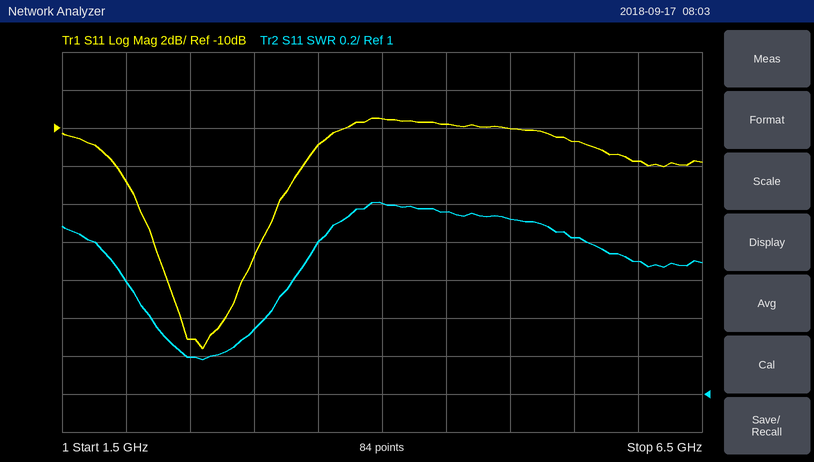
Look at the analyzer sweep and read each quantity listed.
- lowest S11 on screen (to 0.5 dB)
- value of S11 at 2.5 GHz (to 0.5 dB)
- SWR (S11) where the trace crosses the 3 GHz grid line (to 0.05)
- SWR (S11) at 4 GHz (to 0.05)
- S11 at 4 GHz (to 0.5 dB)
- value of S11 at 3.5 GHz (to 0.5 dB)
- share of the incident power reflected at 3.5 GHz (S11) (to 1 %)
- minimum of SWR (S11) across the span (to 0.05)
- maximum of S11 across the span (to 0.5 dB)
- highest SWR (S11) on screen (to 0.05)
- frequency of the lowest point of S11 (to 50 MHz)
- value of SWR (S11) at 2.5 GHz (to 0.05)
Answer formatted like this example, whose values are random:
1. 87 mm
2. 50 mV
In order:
1. -21.5 dB
2. -21.0 dB
3. 1.35
4. 2.00
5. -9.5 dB
6. -11.0 dB
7. 8 %
8. 1.20
9. -9.5 dB
10. 2.00
11. 2.60 GHz
12. 1.20
